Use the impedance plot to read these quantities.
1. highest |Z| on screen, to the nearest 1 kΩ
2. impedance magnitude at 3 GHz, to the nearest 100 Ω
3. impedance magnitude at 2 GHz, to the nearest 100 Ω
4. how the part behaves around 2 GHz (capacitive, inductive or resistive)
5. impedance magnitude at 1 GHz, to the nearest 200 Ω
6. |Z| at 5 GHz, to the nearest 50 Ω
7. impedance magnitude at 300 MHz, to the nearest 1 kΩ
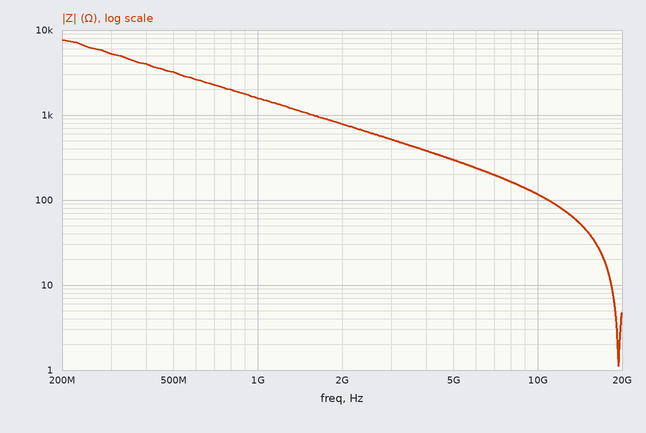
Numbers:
8 kΩ
500 Ω
800 Ω
capacitive
1.6 kΩ
300 Ω
5 kΩ
